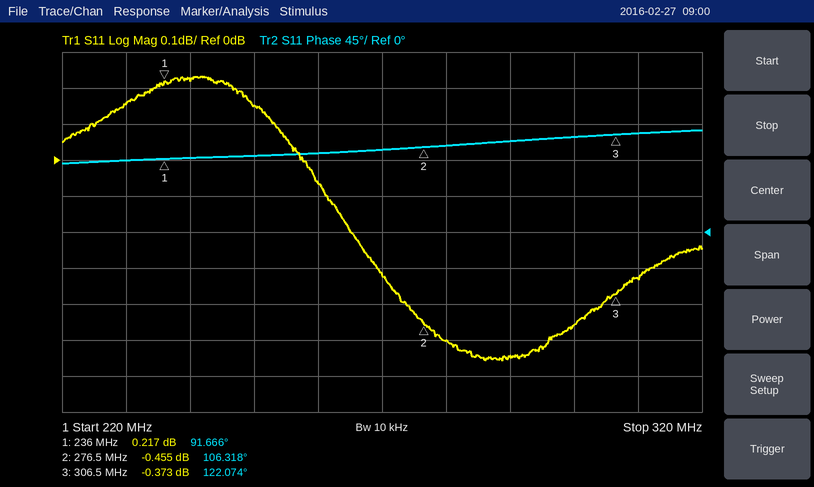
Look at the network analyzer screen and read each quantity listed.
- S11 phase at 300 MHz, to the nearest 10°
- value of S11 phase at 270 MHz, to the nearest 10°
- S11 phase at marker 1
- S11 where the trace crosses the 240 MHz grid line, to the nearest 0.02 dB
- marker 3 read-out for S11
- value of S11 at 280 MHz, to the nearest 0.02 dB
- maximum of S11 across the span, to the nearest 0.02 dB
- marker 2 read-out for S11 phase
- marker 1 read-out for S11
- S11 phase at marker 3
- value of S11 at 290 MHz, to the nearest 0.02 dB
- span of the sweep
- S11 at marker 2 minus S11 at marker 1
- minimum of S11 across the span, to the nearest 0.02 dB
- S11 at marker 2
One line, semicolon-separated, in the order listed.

120°; 100°; 91.666°; 0.22 dB; -0.373 dB; -0.50 dB; 0.24 dB; 106.318°; 0.217 dB; 122.074°; -0.54 dB; 100 MHz; -0.672 dB; -0.56 dB; -0.455 dB
